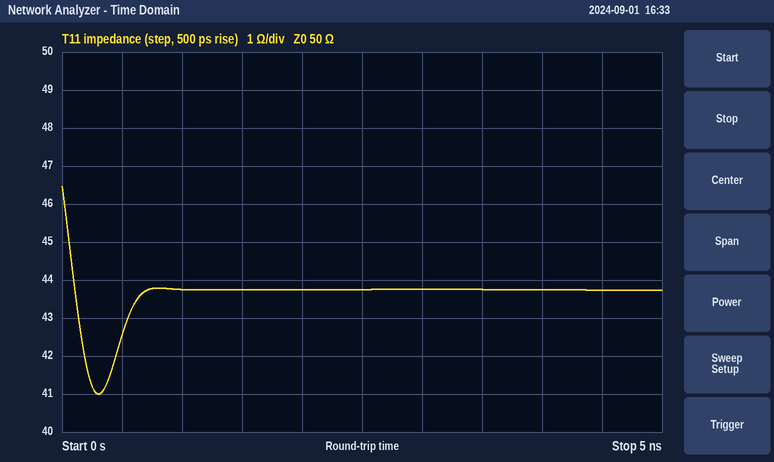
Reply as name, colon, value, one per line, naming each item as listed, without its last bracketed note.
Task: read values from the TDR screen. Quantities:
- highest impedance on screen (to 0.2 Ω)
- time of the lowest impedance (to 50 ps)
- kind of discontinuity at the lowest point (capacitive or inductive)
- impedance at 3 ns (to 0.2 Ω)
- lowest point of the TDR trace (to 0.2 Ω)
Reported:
highest impedance on screen: 46.4 Ω
time of the lowest impedance: 300 ps
kind of discontinuity at the lowest point: capacitive
impedance at 3 ns: 43.8 Ω
lowest point of the TDR trace: 41.0 Ω
